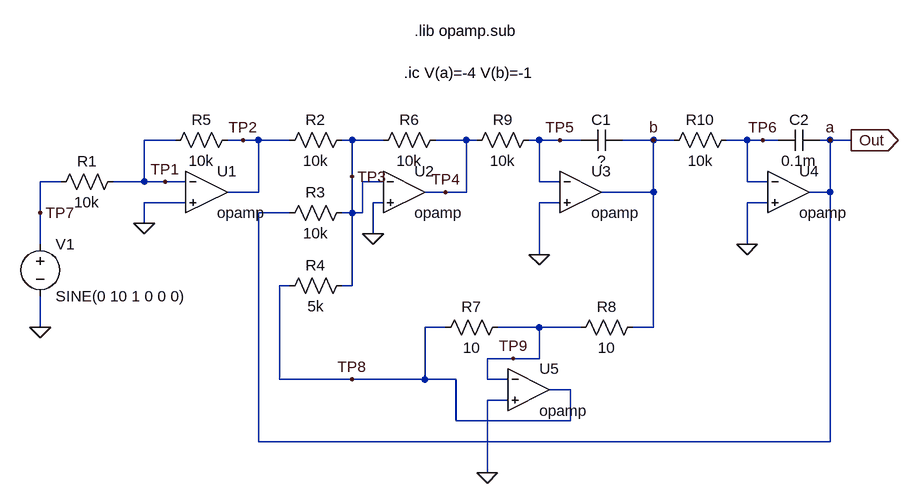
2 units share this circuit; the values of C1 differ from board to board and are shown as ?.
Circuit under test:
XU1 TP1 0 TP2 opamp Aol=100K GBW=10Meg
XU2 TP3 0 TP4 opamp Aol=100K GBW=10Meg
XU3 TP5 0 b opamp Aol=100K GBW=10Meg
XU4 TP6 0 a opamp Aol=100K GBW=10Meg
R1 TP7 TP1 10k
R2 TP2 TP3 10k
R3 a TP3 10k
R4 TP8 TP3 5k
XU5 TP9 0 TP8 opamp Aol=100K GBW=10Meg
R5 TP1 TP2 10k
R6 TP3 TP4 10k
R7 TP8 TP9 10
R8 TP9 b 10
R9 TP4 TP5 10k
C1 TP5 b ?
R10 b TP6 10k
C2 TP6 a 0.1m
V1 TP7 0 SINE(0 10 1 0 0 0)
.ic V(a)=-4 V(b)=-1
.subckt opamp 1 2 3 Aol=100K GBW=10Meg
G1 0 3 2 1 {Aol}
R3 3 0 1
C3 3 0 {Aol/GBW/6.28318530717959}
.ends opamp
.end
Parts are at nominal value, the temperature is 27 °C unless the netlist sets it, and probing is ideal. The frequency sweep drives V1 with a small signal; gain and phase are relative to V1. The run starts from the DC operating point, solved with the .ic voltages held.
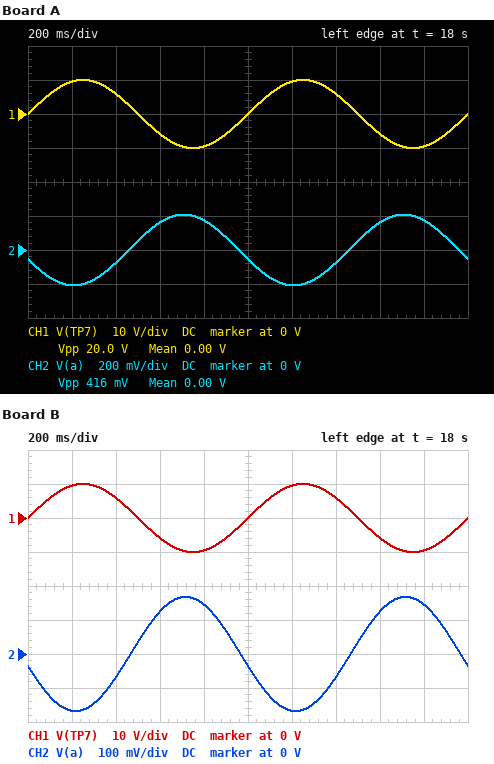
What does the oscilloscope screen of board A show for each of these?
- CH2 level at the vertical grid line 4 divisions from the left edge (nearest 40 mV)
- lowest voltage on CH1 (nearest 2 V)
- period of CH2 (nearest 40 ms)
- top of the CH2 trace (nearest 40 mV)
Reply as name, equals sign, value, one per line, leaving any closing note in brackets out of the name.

CH2 level at the vertical grid line 4 divisions from the left edge = 160 mV
lowest voltage on CH1 = -10 V
period of CH2 = 1.00 s
top of the CH2 trace = 200 mV
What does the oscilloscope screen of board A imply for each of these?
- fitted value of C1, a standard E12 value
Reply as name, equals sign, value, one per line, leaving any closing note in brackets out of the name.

fitted value of C1, a standard E12 value = 120 µF
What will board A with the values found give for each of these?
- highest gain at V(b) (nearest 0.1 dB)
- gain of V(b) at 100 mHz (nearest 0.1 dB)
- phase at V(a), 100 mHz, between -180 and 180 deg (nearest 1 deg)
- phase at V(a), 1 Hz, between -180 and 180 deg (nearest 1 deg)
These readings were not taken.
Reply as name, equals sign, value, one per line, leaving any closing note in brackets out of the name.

highest gain at V(b) = -6.0 dB
gain of V(b) at 100 mHz = -6.7 dB
phase at V(a), 100 mHz, between -180 and 180 deg = -67 deg
phase at V(a), 1 Hz, between -180 and 180 deg = -165 deg
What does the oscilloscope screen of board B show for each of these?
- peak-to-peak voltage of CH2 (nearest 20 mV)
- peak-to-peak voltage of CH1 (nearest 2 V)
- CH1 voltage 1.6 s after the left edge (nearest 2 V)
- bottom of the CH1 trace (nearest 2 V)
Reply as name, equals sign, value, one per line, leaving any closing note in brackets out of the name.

peak-to-peak voltage of CH2 = 340 mV
peak-to-peak voltage of CH1 = 20 V
CH1 voltage 1.6 s after the left edge = -6 V
bottom of the CH1 trace = -10 V
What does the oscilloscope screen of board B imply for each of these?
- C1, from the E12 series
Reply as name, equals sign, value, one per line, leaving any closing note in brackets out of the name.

C1, from the E12 series = 150 µF
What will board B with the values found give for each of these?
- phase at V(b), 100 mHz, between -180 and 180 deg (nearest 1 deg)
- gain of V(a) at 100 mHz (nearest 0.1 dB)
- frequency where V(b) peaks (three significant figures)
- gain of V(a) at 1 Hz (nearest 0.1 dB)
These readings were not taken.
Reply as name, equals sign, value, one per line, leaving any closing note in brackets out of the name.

phase at V(b), 100 mHz, between -180 and 180 deg = -162 deg
gain of V(a) at 100 mHz = -2.4 dB
frequency where V(b) peaks = 130 mHz
gain of V(a) at 1 Hz = -35.5 dB
